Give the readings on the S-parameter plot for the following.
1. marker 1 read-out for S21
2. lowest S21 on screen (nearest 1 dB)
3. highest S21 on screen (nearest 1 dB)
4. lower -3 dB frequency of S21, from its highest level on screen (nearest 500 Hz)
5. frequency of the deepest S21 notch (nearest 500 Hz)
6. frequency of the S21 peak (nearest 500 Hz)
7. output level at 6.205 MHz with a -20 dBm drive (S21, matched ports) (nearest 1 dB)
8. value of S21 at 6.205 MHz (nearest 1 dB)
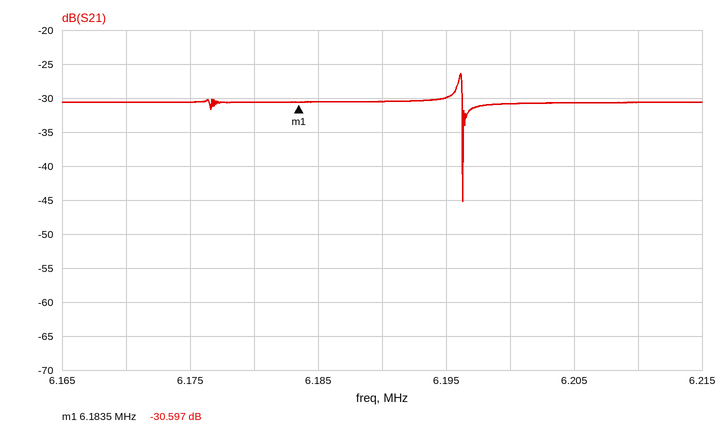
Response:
-30.597 dB
-45 dB
-26 dB
6.1955 MHz
6.1965 MHz
6.1960 MHz
-51 dBm
-31 dB
